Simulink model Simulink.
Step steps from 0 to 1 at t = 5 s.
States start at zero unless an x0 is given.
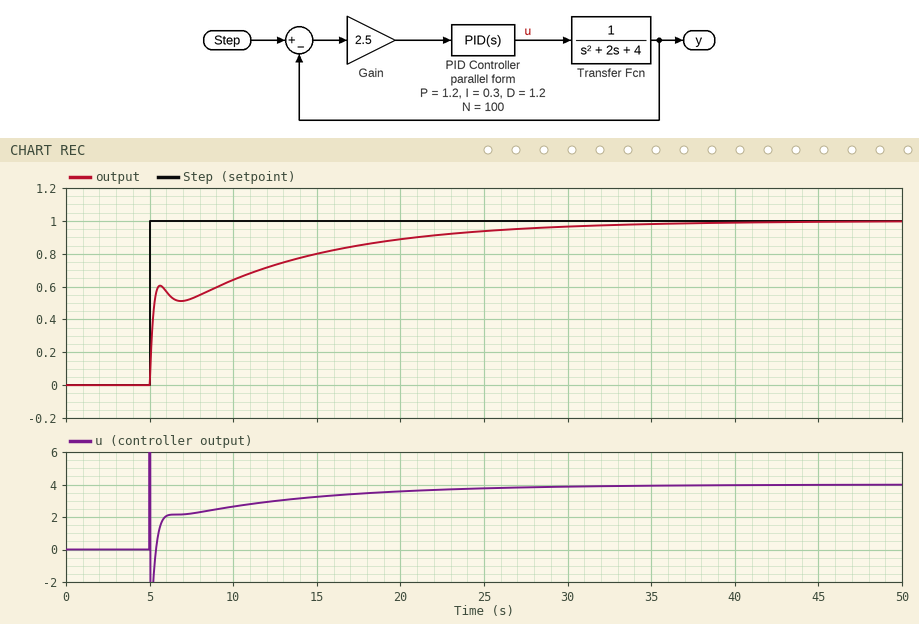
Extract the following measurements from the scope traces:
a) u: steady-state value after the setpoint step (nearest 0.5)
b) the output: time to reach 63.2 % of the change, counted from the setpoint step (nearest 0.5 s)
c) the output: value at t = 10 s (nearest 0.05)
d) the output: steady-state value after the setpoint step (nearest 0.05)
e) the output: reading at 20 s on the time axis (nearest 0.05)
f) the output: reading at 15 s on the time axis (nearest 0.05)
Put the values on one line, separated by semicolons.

4.0; 5.0 s; 0.65; 1.00; 0.90; 0.80
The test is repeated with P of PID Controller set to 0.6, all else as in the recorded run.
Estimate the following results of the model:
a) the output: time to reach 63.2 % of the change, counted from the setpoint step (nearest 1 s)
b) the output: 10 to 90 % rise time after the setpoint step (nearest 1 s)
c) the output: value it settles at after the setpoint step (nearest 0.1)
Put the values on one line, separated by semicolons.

6 s; 14 s; 1.0
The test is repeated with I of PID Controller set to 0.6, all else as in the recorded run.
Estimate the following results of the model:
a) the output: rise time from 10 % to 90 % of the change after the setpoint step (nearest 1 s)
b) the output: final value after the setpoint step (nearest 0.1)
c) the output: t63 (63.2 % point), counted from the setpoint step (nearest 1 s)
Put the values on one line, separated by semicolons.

8 s; 1.0; 3 s
